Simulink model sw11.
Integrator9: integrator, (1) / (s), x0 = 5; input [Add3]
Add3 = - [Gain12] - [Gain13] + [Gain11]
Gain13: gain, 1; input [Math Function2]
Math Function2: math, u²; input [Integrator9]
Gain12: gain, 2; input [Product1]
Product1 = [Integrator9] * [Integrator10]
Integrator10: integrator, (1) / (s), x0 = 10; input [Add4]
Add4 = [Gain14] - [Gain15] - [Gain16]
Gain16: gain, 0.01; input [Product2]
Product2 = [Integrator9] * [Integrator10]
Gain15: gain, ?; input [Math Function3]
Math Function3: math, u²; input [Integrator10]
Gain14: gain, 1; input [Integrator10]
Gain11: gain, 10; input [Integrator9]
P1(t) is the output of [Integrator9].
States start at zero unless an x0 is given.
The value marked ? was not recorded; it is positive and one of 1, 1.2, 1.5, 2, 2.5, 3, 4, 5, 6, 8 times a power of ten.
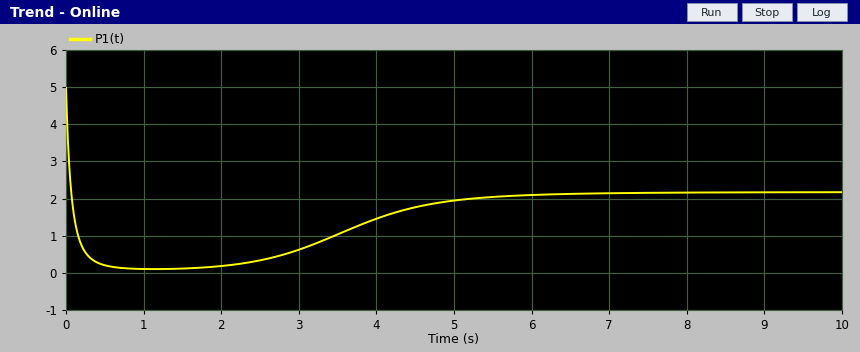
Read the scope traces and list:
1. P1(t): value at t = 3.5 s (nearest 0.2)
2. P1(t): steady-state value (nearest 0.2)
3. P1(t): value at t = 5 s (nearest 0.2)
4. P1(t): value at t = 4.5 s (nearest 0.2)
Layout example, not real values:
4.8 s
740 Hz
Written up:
1.0
2.2
2.0
1.8
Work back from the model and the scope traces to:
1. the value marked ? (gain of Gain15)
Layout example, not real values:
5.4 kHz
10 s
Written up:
0.25
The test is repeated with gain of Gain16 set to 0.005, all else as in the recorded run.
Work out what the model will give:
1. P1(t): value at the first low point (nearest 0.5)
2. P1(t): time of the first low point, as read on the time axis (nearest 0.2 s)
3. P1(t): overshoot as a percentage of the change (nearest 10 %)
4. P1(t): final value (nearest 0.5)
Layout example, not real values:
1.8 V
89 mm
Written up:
0.0
1.2 s
70 %
2.0
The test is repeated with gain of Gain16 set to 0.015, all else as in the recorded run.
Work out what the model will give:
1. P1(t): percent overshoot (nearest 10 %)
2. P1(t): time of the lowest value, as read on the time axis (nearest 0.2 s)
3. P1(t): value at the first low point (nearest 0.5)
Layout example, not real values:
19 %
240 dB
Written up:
80 %
1.2 s
0.0
